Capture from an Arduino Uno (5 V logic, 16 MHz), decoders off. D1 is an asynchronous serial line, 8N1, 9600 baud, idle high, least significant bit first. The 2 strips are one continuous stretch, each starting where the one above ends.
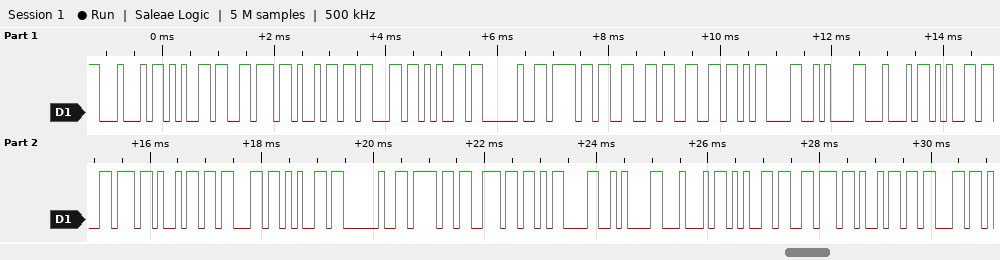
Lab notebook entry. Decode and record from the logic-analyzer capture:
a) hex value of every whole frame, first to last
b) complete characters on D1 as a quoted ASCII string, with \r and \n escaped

44 65 76 69 63 65 20 6F 66 66 0D 0A 44 65 76 69 63 65 20 6F 6E 0D 0A 44 65 76 69 63
"Device off\r\nDevice on\r\nDevic"
